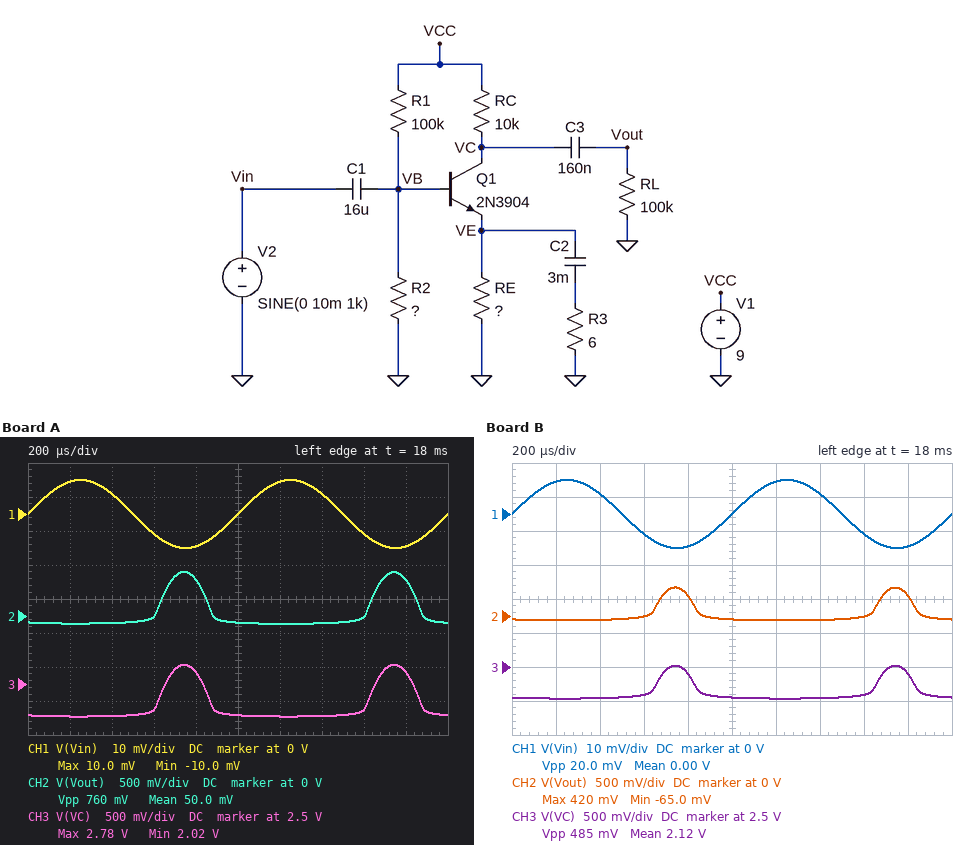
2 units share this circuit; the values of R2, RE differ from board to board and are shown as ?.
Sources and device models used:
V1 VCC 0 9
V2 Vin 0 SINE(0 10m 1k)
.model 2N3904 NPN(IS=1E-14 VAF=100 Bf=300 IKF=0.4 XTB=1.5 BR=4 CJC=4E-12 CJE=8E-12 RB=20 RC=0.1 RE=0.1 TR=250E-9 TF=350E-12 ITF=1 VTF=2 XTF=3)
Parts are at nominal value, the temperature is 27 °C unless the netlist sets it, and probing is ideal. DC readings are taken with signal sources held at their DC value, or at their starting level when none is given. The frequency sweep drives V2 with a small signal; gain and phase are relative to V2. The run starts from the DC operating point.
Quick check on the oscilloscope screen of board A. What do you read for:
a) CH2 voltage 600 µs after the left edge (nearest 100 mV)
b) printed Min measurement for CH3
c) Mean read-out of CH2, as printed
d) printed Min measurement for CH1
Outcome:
0 V
2.02 V
50.0 mV
-10.0 mV
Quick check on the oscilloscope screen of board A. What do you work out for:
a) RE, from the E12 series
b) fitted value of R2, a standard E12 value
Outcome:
2.7 kΩ
120 kΩ
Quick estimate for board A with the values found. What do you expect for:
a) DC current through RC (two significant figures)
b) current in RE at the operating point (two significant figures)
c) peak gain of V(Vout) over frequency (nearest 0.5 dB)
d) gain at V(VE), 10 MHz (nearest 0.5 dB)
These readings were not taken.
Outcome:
700 µA
740 µA
9.5 dB
-19.5 dB
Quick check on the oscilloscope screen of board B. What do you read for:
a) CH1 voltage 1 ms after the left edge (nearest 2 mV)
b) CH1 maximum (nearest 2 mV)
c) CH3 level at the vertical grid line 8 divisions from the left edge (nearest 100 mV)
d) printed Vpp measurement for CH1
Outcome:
0 V
10 mV
2.1 V
20.0 mV
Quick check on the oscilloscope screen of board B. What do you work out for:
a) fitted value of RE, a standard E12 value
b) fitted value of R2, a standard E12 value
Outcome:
2.7 kΩ
180 kΩ
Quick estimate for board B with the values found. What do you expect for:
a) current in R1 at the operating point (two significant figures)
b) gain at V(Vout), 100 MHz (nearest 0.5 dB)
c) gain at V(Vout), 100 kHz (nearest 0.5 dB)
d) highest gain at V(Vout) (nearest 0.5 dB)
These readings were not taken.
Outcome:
63 µA
-4.0 dB
8.0 dB
8.0 dB
